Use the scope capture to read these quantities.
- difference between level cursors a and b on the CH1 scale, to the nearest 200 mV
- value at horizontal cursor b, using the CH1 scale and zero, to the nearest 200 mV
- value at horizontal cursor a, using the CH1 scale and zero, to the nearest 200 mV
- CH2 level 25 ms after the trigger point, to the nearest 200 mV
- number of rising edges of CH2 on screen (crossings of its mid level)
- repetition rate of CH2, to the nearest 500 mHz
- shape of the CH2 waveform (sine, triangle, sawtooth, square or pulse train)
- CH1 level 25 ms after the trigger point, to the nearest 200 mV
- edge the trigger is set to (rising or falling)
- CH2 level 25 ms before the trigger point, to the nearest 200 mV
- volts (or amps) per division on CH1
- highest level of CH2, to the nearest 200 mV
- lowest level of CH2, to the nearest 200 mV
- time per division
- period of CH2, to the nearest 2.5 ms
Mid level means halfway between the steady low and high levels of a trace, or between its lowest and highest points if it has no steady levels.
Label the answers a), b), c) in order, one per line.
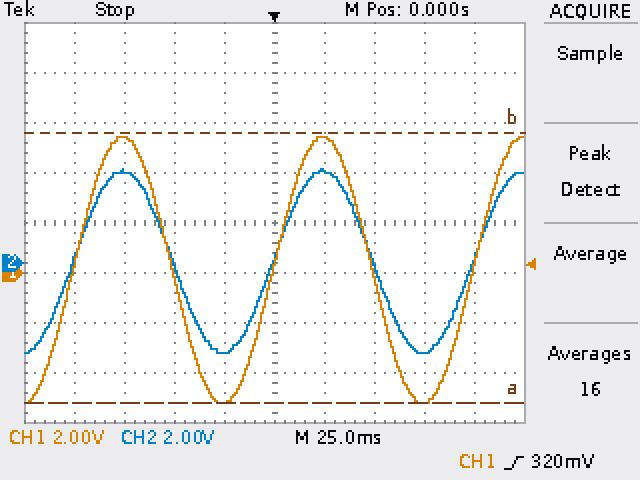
a) 10.8 V
b) 5.6 V
c) -5.2 V
d) 3.6 V
e) 3
f) 10.0 Hz
g) sine
h) 5.4 V
i) rising
j) -3.6 V
k) 2 V
l) 3.8 V
m) -3.6 V
n) 25 ms
o) 100.0 ms
